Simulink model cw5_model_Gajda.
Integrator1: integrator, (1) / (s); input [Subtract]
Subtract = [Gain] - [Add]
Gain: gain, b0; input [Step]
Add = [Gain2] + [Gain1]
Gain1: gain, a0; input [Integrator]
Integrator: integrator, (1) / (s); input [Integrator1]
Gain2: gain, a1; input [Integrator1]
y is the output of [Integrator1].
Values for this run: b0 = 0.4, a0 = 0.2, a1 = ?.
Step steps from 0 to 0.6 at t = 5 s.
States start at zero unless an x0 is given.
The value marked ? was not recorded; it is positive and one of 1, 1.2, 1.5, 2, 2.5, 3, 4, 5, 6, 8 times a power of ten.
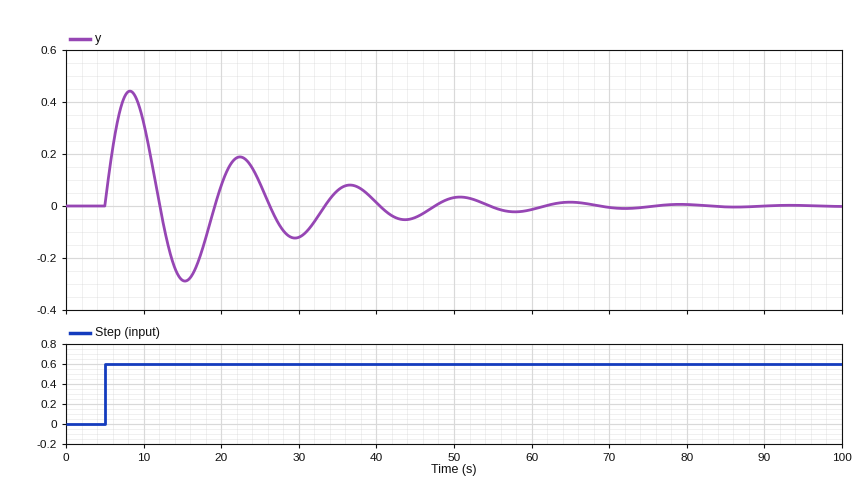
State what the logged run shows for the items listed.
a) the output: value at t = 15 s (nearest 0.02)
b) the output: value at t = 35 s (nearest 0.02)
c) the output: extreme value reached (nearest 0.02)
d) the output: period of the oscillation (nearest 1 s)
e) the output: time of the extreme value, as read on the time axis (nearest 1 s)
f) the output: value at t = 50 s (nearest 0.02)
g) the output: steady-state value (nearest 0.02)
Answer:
-0.28
0.06
0.44
14 s
8 s
0.04
0.00
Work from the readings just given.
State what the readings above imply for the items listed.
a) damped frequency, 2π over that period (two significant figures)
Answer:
0.45 rad/s
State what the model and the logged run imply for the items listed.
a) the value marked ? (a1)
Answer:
0.12
